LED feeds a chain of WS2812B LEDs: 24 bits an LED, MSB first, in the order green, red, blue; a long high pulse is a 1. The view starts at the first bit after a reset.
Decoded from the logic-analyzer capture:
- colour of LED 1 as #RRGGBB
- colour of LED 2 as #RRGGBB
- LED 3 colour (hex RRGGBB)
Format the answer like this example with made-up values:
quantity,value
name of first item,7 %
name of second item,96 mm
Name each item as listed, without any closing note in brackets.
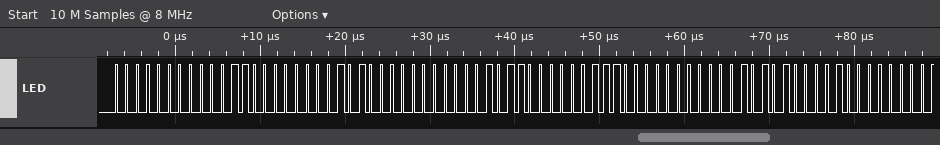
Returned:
quantity,value
colour of LED 1 as #RRGGBB,#180005
colour of LED 2 as #RRGGBB,#160007
LED 3 colour,#150008
